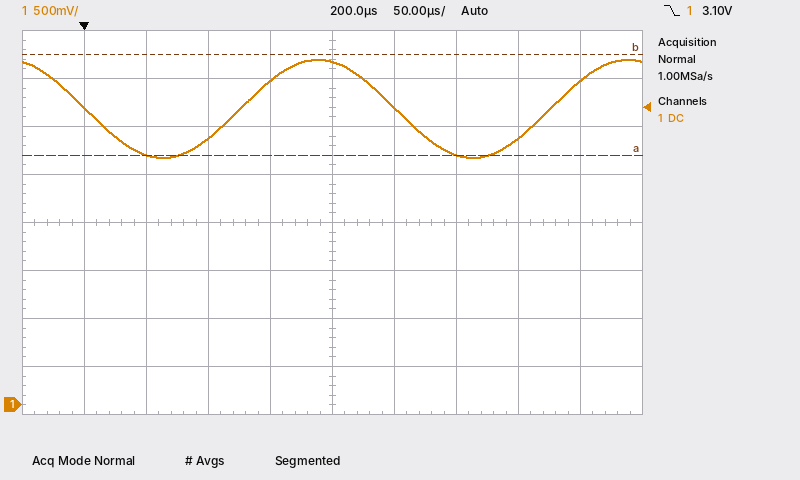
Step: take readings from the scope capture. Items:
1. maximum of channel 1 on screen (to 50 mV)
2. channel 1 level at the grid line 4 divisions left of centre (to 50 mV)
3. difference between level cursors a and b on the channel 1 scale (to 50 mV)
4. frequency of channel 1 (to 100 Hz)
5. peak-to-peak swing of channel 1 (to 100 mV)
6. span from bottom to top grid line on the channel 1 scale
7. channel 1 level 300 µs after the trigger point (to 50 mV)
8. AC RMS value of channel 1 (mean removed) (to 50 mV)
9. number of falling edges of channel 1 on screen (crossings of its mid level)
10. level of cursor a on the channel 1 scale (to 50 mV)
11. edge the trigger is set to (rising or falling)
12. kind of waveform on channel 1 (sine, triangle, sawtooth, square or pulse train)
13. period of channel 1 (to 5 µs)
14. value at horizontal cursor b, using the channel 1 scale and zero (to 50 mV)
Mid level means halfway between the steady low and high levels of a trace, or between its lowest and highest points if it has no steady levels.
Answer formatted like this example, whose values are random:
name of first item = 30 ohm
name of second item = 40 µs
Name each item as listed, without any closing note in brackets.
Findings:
maximum of channel 1 on screen = 3.60 V
channel 1 level at the grid line 4 divisions left of centre = 3.10 V
difference between level cursors a and b on the channel 1 scale = 1.05 V
frequency of channel 1 = 4.0 kHz
peak-to-peak swing of channel 1 = 1.00 V
span from bottom to top grid line on the channel 1 scale = 4 V
channel 1 level 300 µs after the trigger point = 2.60 V
AC RMS value of channel 1 (mean removed) = 350 mV
number of falling edges of channel 1 on screen = 2
level of cursor a on the channel 1 scale = 2.60 V
edge the trigger is set to = falling
kind of waveform on channel 1 = sine
period of channel 1 = 250 µs
value at horizontal cursor b, using the channel 1 scale and zero = 3.65 V
